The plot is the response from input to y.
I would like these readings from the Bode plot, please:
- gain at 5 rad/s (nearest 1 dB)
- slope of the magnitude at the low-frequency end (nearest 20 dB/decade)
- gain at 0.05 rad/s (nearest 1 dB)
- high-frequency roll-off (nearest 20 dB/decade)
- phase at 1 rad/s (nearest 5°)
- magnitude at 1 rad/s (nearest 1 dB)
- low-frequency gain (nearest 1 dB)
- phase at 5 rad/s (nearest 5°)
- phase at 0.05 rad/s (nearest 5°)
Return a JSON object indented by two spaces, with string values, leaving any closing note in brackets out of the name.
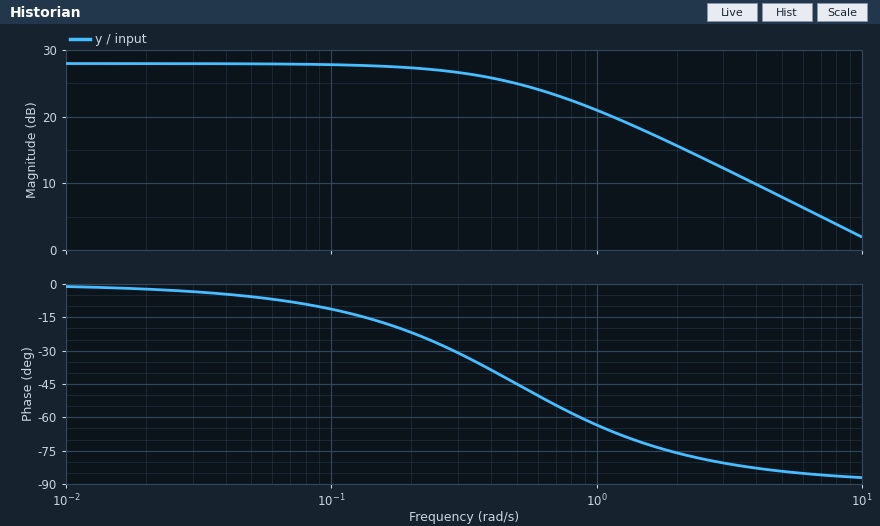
{
  "gain at 5 rad/s": "8 dB",
  "slope of the magnitude at the low-frequency end": "0 dB/decade",
  "gain at 0.05 rad/s": "28 dB",
  "high-frequency roll-off": "-20 dB/decade",
  "phase at 1 rad/s": "-65°",
  "magnitude at 1 rad/s": "21 dB",
  "low-frequency gain": "28 dB",
  "phase at 5 rad/s": "-85°",
  "phase at 0.05 rad/s": "-5°"
}
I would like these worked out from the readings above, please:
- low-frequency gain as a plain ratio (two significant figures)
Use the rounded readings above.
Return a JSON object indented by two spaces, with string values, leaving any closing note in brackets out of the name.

{
  "low-frequency gain as a plain ratio": "25"
}
